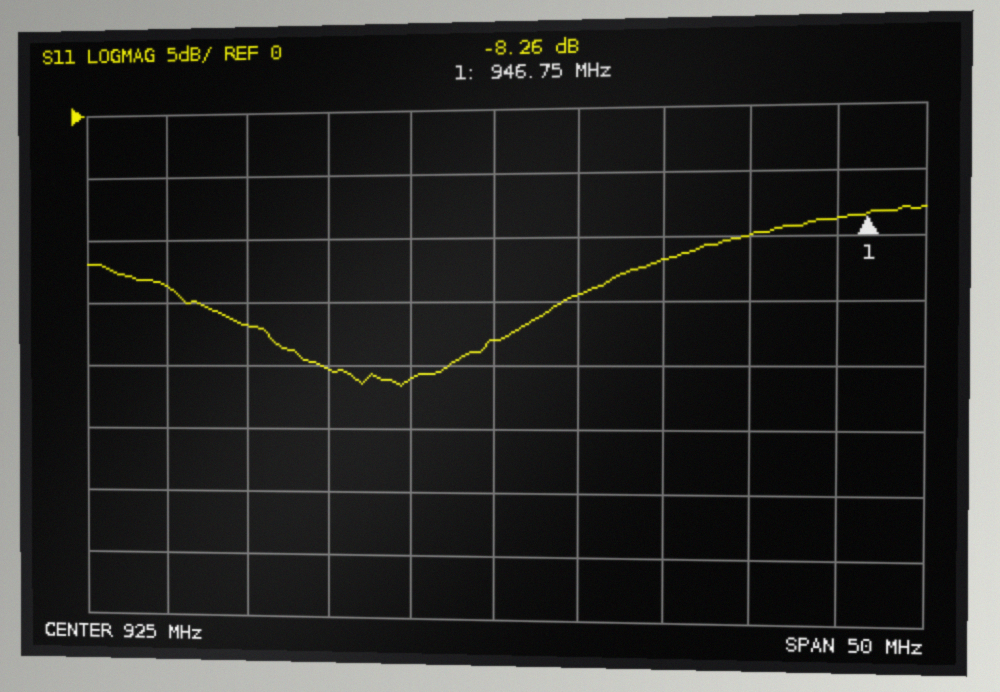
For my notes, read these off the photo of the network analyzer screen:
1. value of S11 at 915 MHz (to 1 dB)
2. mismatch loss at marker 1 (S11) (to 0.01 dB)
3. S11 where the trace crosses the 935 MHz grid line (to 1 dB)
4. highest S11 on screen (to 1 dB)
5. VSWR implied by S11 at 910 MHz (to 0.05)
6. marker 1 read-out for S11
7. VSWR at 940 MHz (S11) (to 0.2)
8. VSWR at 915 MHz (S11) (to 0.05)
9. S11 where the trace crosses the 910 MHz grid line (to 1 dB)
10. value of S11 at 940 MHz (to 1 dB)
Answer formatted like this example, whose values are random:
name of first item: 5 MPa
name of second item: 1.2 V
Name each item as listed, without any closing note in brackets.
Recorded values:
value of S11 at 915 MHz: -20 dB
mismatch loss at marker 1 (S11): 0.70 dB
S11 where the trace crosses the 935 MHz grid line: -12 dB
highest S11 on screen: -8 dB
VSWR implied by S11 at 910 MHz: 1.35
marker 1 read-out for S11: -8.26 dB
VSWR at 940 MHz (S11): 2.0
VSWR at 915 MHz (S11): 1.20
S11 where the trace crosses the 910 MHz grid line: -17 dB
value of S11 at 940 MHz: -10 dB
